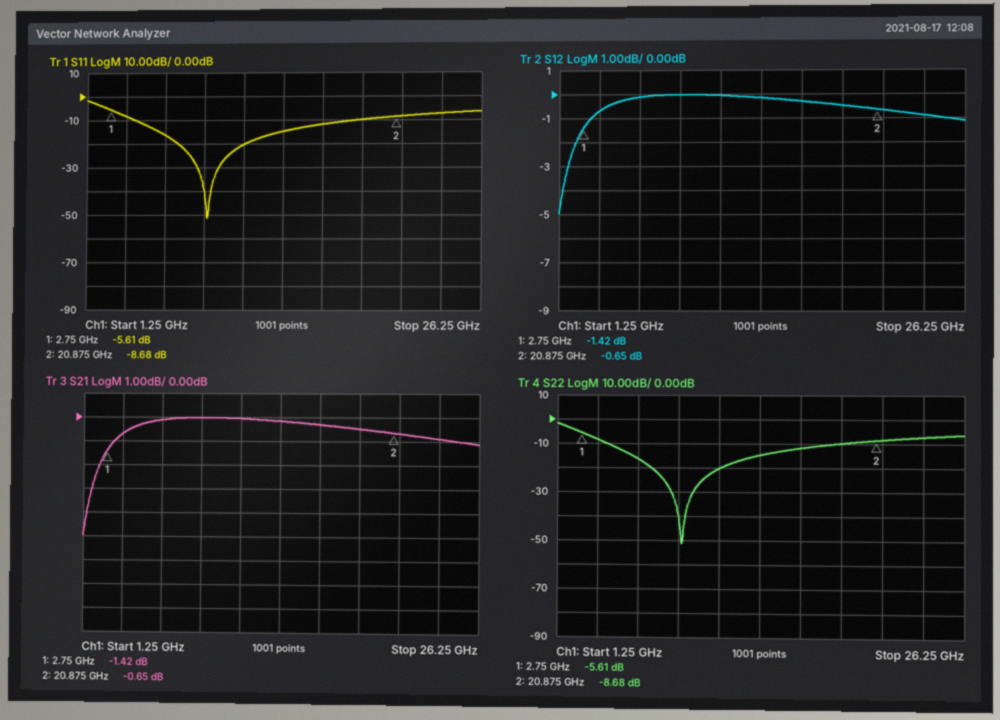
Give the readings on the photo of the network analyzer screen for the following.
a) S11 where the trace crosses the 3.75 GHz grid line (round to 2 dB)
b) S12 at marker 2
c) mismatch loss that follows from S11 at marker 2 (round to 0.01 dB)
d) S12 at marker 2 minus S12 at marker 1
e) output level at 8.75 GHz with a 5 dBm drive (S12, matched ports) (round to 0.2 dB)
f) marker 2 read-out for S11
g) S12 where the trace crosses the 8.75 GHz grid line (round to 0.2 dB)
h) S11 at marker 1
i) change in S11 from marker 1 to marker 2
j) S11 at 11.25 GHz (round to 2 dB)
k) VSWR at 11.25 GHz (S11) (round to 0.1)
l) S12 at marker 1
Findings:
-8 dB
-0.65 dB
0.63 dB
0.77 dB
5.0 dBm
-8.68 dB
0.0 dB
-5.61 dB
-3.07 dB
-20 dB
1.2
-1.42 dB
